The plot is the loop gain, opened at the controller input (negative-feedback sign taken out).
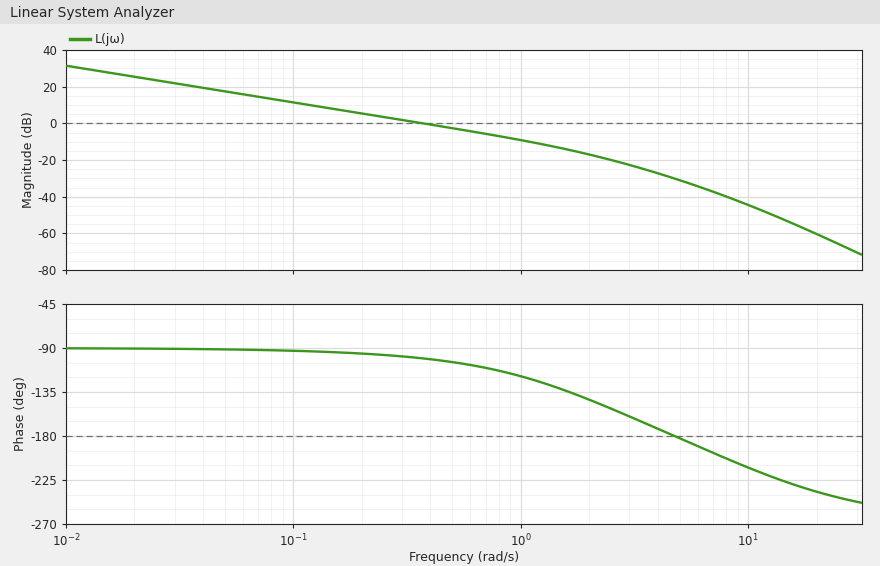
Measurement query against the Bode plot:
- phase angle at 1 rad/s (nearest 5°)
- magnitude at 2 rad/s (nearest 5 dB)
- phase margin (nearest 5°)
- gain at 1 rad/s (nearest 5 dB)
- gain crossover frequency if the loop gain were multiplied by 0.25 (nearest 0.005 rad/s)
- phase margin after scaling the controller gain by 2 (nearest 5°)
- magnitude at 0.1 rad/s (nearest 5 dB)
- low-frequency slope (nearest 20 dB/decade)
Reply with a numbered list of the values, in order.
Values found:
1. -120°
2. -15 dB
3. 80°
4. -10 dB
5. 0.095 rad/s
6. 70°
7. 10 dB
8. -20 dB/decade
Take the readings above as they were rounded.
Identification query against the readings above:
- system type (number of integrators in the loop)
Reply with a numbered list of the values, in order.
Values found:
1. 1
